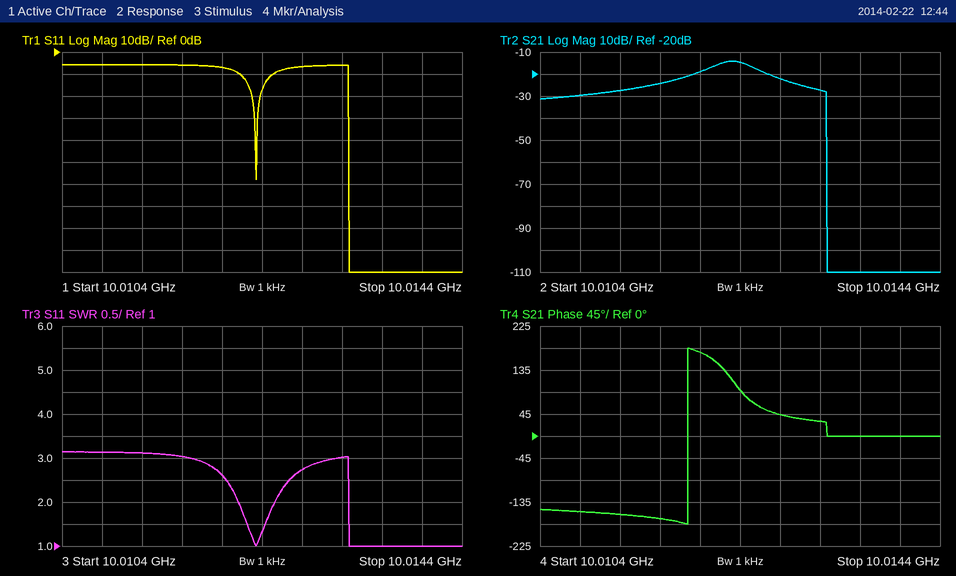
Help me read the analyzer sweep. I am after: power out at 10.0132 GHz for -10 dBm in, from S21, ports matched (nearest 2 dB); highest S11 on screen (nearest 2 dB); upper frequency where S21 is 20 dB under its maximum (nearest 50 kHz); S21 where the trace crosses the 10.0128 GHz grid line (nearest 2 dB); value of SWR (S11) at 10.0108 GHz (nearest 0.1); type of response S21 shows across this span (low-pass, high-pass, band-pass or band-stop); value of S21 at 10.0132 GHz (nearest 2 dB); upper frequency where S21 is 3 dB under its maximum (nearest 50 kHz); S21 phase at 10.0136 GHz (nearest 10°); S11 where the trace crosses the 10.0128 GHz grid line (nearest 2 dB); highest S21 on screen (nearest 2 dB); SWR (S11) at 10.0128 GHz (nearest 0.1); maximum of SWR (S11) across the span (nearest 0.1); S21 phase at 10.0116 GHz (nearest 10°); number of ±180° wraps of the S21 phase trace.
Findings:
-38 dBm
-6 dB
10.01325 GHz
-22 dB
3.1
band-pass
-28 dB
10.01255 GHz
0°
-6 dB
-14 dB
2.7
3.1
-170°
1
